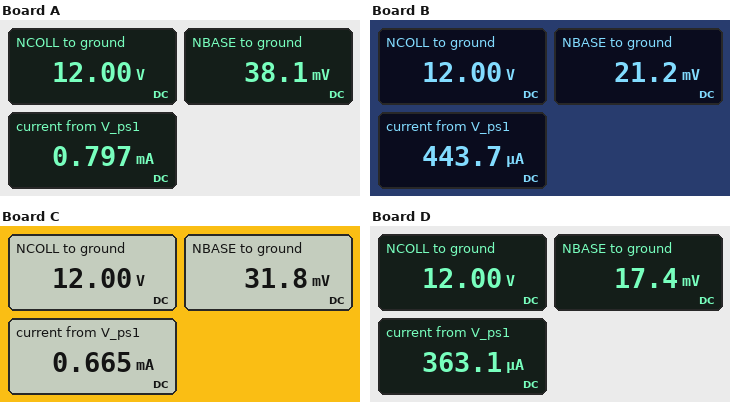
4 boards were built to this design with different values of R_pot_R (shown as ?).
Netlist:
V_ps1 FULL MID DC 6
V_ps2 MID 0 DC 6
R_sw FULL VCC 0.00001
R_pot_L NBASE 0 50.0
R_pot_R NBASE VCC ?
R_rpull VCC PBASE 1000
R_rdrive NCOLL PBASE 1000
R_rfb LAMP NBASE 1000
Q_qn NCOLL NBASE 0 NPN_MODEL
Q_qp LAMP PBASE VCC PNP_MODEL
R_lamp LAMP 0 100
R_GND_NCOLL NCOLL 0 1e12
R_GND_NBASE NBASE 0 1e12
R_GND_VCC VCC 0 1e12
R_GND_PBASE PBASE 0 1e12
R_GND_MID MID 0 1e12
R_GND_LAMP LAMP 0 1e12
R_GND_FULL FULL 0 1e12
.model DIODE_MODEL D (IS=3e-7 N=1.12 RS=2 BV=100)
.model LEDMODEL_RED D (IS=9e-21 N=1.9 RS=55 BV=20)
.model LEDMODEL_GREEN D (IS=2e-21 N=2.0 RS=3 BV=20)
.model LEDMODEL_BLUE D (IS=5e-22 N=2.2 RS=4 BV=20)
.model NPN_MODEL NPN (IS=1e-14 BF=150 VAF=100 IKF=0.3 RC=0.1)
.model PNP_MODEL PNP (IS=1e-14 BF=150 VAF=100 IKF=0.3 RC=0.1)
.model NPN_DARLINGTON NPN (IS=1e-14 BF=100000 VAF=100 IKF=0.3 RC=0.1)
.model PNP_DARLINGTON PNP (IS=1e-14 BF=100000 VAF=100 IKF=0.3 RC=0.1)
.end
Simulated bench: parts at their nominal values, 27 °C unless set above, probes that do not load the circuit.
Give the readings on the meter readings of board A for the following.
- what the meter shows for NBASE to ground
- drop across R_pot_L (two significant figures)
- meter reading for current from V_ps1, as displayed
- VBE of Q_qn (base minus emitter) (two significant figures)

38.1 mV
38 mV
0.797 mA
38 mV
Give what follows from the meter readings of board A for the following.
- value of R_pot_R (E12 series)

15 kΩ
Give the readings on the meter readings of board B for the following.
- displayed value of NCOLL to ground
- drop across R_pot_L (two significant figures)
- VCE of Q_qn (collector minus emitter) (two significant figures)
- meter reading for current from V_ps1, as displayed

12.00 V
21 mV
12 V
443.7 µA
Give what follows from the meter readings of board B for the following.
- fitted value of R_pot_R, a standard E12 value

27 kΩ
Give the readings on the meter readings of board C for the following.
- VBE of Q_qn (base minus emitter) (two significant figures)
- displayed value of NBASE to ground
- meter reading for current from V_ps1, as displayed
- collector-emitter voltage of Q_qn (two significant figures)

32 mV
31.8 mV
0.665 mA
12 V
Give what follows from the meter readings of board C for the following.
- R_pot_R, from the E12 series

18 kΩ
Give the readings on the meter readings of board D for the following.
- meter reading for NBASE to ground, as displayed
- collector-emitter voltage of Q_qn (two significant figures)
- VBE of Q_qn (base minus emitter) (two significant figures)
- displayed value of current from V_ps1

17.4 mV
12 V
17 mV
363.1 µA
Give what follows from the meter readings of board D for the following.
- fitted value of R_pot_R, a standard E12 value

33 kΩ
